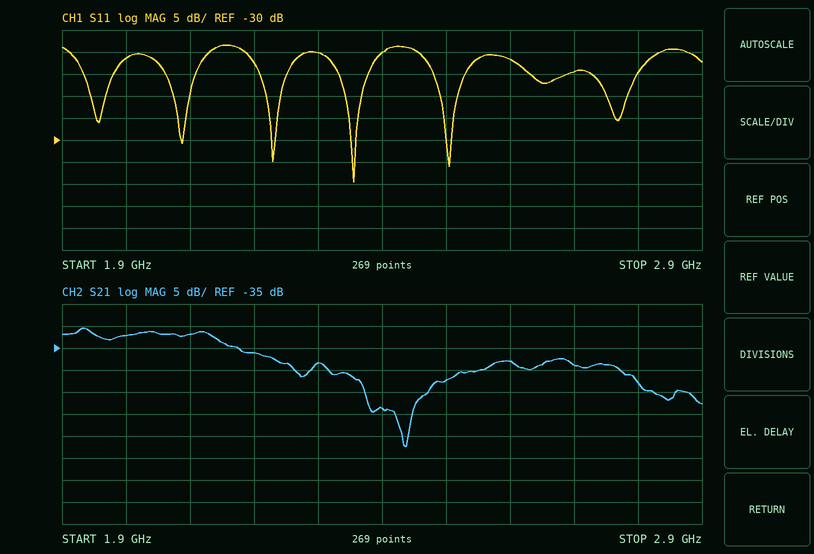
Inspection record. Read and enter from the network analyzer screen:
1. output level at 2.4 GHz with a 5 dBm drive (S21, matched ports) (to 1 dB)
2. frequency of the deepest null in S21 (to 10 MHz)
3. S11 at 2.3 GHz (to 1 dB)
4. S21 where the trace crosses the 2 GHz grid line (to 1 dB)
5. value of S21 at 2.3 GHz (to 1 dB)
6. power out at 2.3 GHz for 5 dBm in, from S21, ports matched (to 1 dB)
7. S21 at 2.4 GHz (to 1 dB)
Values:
-44 dBm
2.44 GHz
-10 dB
-32 dB
-38 dB
-33 dBm
-49 dB
